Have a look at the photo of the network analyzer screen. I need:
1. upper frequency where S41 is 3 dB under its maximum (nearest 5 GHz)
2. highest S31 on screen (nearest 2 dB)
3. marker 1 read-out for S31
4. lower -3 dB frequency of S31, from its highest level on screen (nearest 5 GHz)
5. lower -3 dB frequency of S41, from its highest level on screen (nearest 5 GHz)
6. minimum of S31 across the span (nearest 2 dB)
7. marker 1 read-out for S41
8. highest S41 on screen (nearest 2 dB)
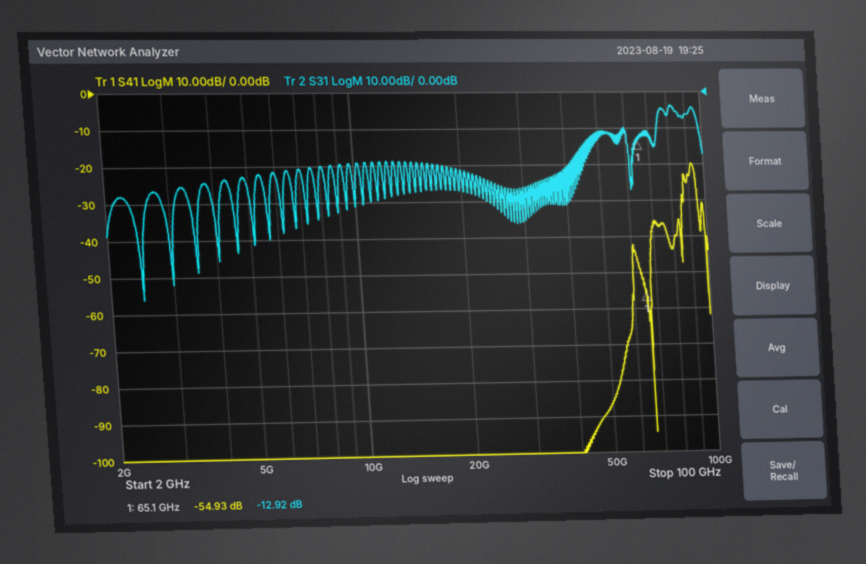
95 GHz
-4 dB
-12.92 dB
75 GHz
90 GHz
-56 dB
-54.93 dB
-20 dB
